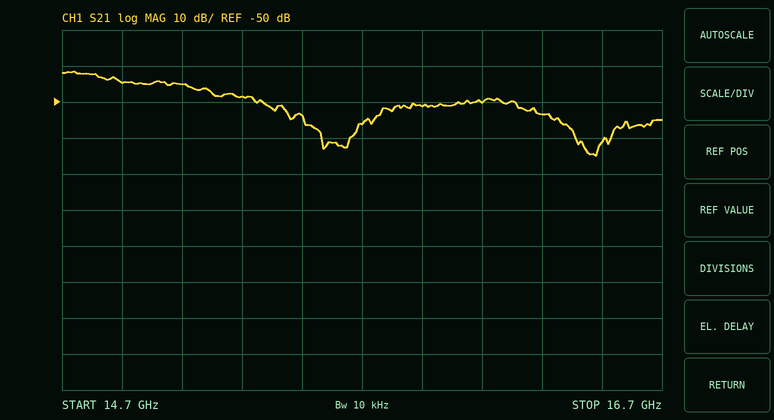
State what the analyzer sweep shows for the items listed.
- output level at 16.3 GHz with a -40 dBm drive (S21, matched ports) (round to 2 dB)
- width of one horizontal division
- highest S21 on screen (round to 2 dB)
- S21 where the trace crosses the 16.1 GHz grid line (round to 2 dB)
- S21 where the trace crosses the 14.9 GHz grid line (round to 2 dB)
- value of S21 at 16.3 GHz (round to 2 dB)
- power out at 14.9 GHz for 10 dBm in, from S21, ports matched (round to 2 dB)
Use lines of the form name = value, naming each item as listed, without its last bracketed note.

output level at 16.3 GHz with a -40 dBm drive (S21, matched ports) = -94 dBm
width of one horizontal division = 200 MHz
highest S21 on screen = -42 dB
S21 where the trace crosses the 16.1 GHz grid line = -50 dB
S21 where the trace crosses the 14.9 GHz grid line = -44 dB
value of S21 at 16.3 GHz = -54 dB
power out at 14.9 GHz for 10 dBm in, from S21, ports matched = -34 dBm
